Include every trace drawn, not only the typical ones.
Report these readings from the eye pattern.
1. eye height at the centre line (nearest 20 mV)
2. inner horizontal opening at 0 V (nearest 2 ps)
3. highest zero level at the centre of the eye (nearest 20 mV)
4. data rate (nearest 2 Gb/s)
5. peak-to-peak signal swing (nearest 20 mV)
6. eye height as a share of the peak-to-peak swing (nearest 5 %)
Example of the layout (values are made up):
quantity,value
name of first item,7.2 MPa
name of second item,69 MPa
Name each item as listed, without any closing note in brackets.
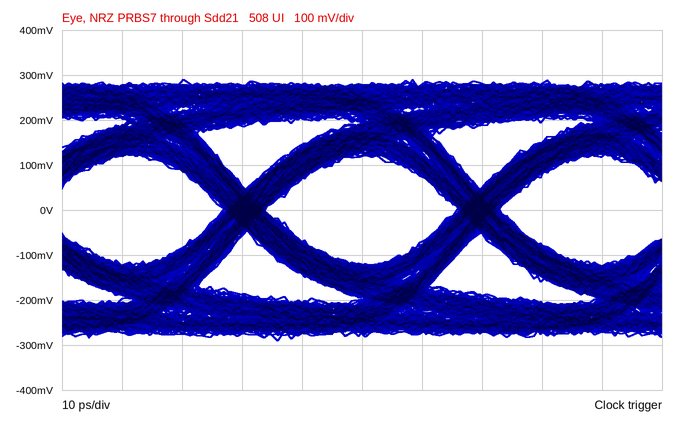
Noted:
quantity,value
eye height at the centre line,240 mV
inner horizontal opening at 0 V,32 ps
highest zero level at the centre of the eye,-120 mV
data rate,26 Gb/s
peak-to-peak signal swing,580 mV
eye height as a share of the peak-to-peak swing,40 %
